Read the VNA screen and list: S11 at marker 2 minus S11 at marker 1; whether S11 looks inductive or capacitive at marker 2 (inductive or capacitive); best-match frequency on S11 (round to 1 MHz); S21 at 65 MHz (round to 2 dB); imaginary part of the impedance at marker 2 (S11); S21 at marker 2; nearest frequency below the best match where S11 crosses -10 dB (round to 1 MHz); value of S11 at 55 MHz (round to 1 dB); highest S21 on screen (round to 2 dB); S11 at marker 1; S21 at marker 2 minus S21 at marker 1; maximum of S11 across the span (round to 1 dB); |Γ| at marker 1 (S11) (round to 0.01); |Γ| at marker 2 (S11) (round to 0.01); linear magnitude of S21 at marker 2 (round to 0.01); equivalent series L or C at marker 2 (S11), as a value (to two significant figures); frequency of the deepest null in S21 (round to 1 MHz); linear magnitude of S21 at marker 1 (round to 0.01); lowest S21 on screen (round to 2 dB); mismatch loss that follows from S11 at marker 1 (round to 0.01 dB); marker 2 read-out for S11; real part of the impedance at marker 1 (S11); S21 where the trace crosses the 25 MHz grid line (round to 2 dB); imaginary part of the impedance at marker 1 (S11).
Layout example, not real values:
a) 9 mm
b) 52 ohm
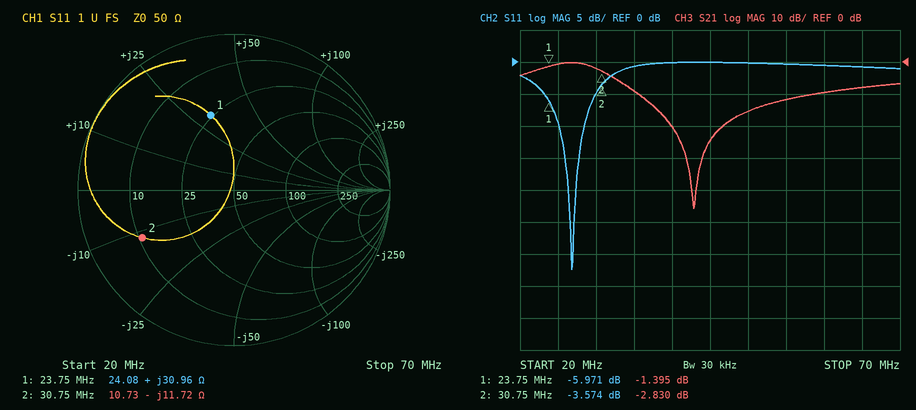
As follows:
a) 2.397 dB
b) capacitive
c) 27 MHz
d) -8 dB
e) -11.72 Ω
f) -2.830 dB
g) 25 MHz
h) 0 dB
i) 0 dB
j) -5.971 dB
k) -1.435 dB
l) 0 dB
m) 0.50
n) 0.66
o) 0.72
p) 440 pF
q) 43 MHz
r) 0.85
s) -46 dB
t) 1.27 dB
u) -3.574 dB
v) 24.08 Ω
w) 0 dB
x) +30.96 Ω
